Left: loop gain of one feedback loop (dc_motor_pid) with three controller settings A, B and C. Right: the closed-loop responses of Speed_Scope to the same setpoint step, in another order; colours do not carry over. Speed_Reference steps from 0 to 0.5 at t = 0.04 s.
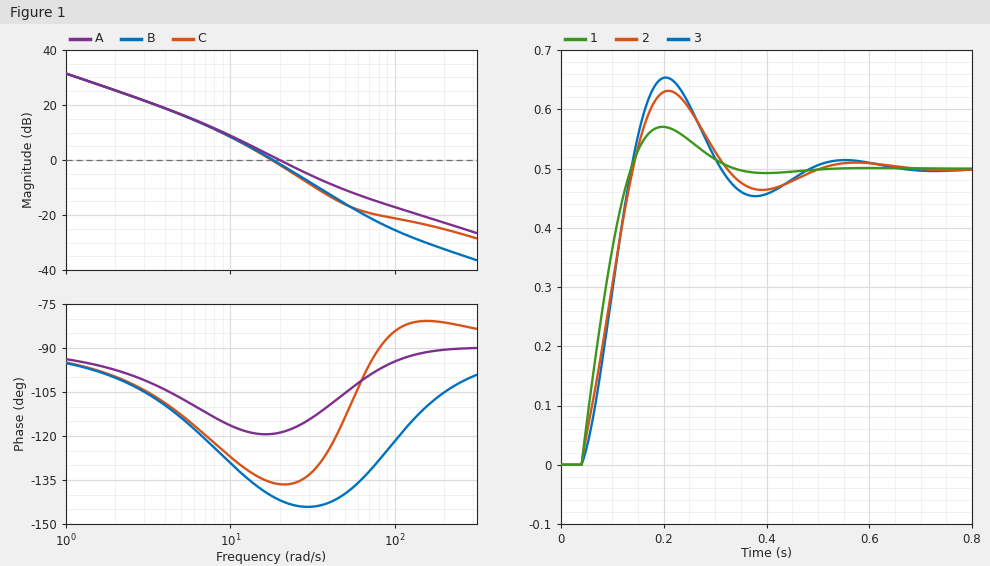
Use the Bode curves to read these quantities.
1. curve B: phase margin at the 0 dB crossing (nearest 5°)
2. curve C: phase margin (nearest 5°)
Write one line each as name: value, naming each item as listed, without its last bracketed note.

curve B: phase margin at the 0 dB crossing: 40°
curve C: phase margin: 45°
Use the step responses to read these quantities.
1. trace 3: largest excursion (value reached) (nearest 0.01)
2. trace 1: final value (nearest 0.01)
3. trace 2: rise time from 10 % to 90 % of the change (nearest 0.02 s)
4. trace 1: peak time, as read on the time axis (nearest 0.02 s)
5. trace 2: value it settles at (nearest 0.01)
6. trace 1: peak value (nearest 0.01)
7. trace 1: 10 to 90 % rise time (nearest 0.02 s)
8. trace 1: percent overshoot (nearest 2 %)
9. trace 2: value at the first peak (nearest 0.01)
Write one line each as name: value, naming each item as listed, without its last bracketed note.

trace 3: largest excursion (value reached): 0.65
trace 1: final value: 0.50
trace 2: rise time from 10 % to 90 % of the change: 0.08 s
trace 1: peak time, as read on the time axis: 0.20 s
trace 2: value it settles at: 0.50
trace 1: peak value: 0.57
trace 1: 10 to 90 % rise time: 0.08 s
trace 1: percent overshoot: 14 %
trace 2: value at the first peak: 0.63
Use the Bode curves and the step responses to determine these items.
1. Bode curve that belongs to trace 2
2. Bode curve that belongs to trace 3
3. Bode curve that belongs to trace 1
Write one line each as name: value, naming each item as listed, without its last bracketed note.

Bode curve that belongs to trace 2: C
Bode curve that belongs to trace 3: B
Bode curve that belongs to trace 1: A
